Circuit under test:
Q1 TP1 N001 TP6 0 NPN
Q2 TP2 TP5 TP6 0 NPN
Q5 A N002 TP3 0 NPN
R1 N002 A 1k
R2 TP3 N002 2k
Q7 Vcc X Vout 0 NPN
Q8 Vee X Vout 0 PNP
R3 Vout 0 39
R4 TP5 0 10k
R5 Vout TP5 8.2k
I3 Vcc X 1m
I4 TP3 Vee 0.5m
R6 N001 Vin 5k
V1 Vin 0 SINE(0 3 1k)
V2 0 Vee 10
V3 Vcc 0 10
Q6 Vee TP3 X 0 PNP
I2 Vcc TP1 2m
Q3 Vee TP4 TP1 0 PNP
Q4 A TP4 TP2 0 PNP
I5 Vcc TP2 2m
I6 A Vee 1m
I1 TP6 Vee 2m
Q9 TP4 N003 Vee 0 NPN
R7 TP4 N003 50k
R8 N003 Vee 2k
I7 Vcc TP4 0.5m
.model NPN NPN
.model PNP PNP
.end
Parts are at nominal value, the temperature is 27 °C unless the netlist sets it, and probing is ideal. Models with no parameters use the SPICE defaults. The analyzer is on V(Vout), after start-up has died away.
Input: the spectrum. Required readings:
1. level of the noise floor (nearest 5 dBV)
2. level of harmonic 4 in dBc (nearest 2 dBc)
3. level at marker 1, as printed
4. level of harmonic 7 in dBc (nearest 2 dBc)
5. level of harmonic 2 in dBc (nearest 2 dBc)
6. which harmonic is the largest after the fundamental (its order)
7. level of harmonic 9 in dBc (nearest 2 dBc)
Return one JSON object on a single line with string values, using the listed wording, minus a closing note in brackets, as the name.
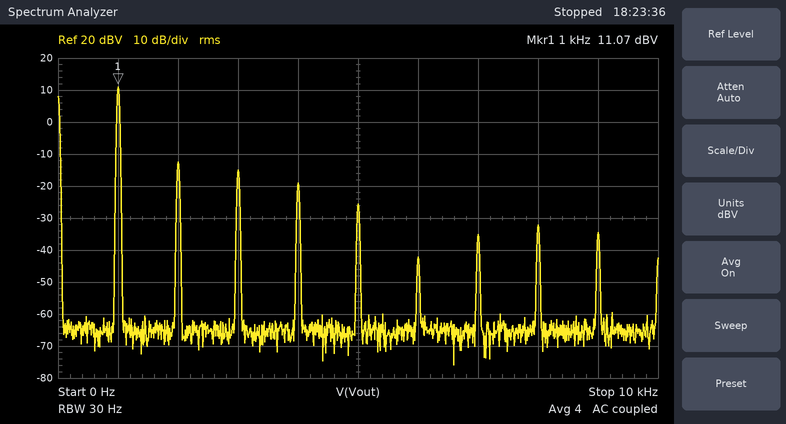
{"level of the noise floor": "-65 dBV", "level of harmonic 4 in dBc": "-30 dBc", "level at marker 1, as printed": "11.07 dBV", "level of harmonic 7 in dBc": "-46 dBc", "level of harmonic 2 in dBc": "-24 dBc", "which harmonic is the largest after the fundamental": "2", "level of harmonic 9 in dBc": "-46 dBc"}
